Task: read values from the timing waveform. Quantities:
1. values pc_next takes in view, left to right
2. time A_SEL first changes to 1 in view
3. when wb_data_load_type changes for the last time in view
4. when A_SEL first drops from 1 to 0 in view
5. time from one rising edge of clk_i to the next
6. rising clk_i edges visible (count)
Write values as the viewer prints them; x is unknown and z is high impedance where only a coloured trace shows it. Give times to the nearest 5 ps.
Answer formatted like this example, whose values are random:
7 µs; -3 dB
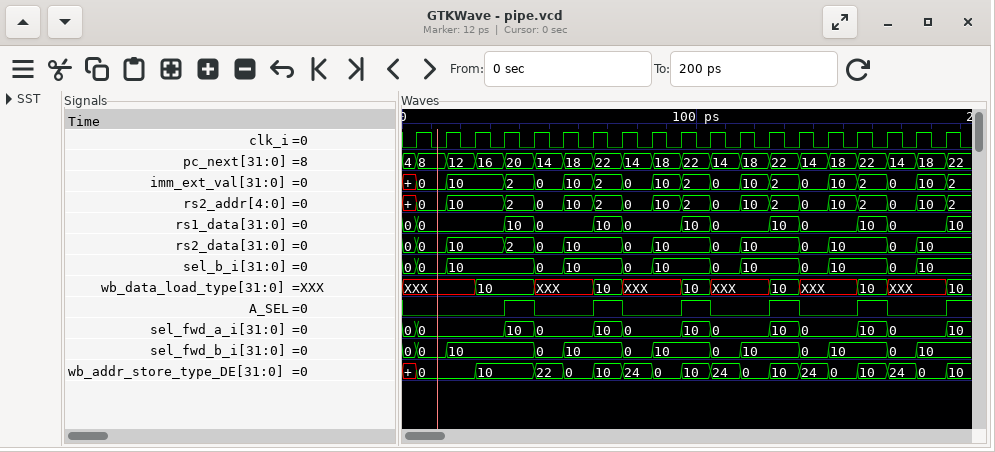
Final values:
4, 8, 12, 16, 20, 14, 18, 22, 14, 18, 22, 14, 18, 22, 14, 18, 22, 14, 18, 22; 35 ps; 185 ps; 45 ps; 10 ps; 19
